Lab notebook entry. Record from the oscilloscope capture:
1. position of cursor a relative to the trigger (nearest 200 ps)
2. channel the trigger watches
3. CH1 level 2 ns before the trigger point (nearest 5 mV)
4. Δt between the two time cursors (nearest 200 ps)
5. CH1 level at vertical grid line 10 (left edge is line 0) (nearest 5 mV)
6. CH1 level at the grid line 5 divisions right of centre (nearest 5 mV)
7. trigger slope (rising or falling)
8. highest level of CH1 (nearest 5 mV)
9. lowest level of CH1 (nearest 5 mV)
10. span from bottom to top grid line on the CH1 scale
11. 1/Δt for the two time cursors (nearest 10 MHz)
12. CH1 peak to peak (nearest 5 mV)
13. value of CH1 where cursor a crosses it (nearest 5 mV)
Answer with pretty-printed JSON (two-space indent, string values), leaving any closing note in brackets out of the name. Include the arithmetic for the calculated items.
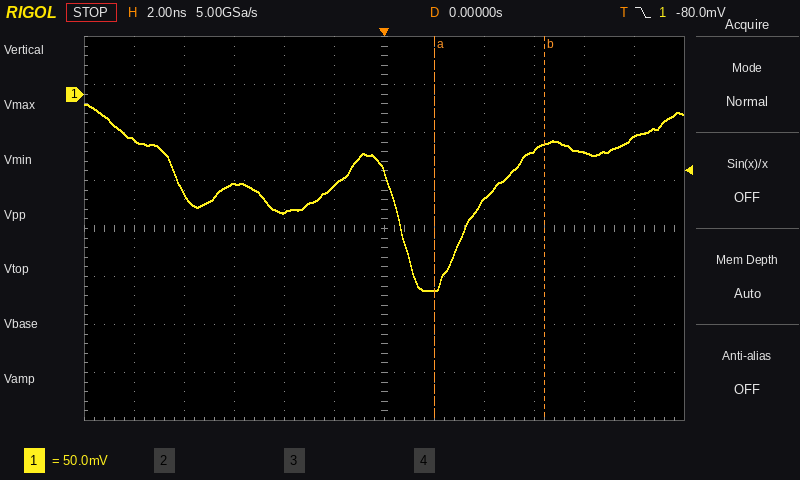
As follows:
{
  "position of cursor a relative to the trigger": "+2.0 ns",
  "channel the trigger watches": "CH1",
  "CH1 level 2 ns before the trigger point": "-95 mV",
  "Δt between the two time cursors": "4.4 ns",
  "CH1 level at vertical grid line 10 (left edge is line 0)": "-60 mV",
  "CH1 level at the grid line 5 divisions right of centre": "-45 mV",
  "trigger slope": "falling",
  "highest level of CH1": "-10 mV",
  "lowest level of CH1": "-205 mV",
  "span from bottom to top grid line on the CH1 scale": "400 mV",
  "1/Δt for the two time cursors": "1 / 4.4 ns ≈ 230 MHz",
  "CH1 peak to peak": "-10 mV − (-205 mV) = 195 mV",
  "value of CH1 where cursor a crosses it": "-205 mV"
}
